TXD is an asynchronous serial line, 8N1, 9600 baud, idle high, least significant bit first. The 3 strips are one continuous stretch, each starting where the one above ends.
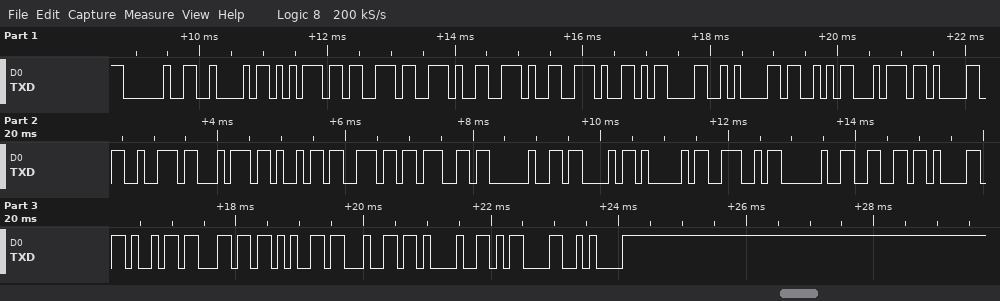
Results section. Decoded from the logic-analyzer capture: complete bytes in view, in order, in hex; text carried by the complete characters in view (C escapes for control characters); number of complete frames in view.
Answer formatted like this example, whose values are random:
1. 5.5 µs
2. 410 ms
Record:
1. 20 42 75 73 2E 2E 2E 0D 0A 53 74 61 72 74 69 6E 67 20 43 41 4E 20 66 61 69 6C 65 64 21 0D 0A
2. " Bus...\r\nStarting CAN failed!\r\n"
3. 31
